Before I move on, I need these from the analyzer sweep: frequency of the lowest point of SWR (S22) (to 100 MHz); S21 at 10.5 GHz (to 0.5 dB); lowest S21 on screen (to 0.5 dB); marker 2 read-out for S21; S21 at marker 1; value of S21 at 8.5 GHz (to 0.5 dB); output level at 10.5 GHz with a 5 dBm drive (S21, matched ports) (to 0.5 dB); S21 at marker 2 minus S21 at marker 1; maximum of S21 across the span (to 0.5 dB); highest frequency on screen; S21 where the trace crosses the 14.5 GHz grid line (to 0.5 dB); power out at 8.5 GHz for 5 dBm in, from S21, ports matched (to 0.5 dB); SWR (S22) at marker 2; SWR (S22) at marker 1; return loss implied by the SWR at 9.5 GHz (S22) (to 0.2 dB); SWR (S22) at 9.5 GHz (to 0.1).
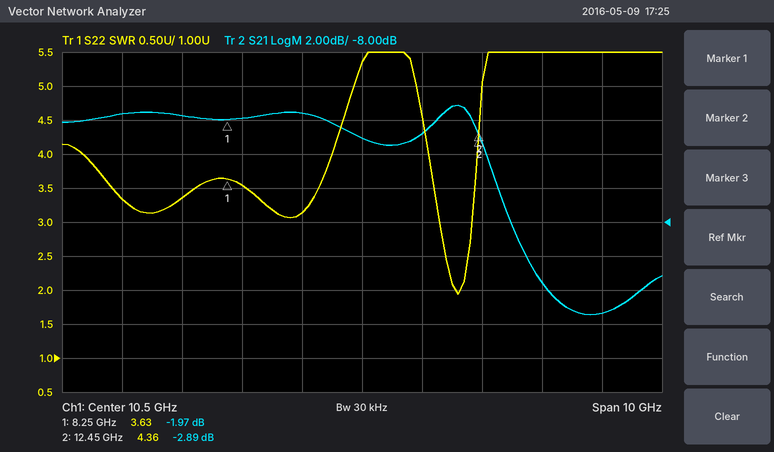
12.1 GHz
-3.0 dB
-13.5 dB
-2.89 dB
-1.97 dB
-2.0 dB
2.0 dBm
-0.92 dB
-1.0 dB
15.5 GHz
-13.5 dB
3.0 dBm
4.36
3.63
5.8 dB
3.1
